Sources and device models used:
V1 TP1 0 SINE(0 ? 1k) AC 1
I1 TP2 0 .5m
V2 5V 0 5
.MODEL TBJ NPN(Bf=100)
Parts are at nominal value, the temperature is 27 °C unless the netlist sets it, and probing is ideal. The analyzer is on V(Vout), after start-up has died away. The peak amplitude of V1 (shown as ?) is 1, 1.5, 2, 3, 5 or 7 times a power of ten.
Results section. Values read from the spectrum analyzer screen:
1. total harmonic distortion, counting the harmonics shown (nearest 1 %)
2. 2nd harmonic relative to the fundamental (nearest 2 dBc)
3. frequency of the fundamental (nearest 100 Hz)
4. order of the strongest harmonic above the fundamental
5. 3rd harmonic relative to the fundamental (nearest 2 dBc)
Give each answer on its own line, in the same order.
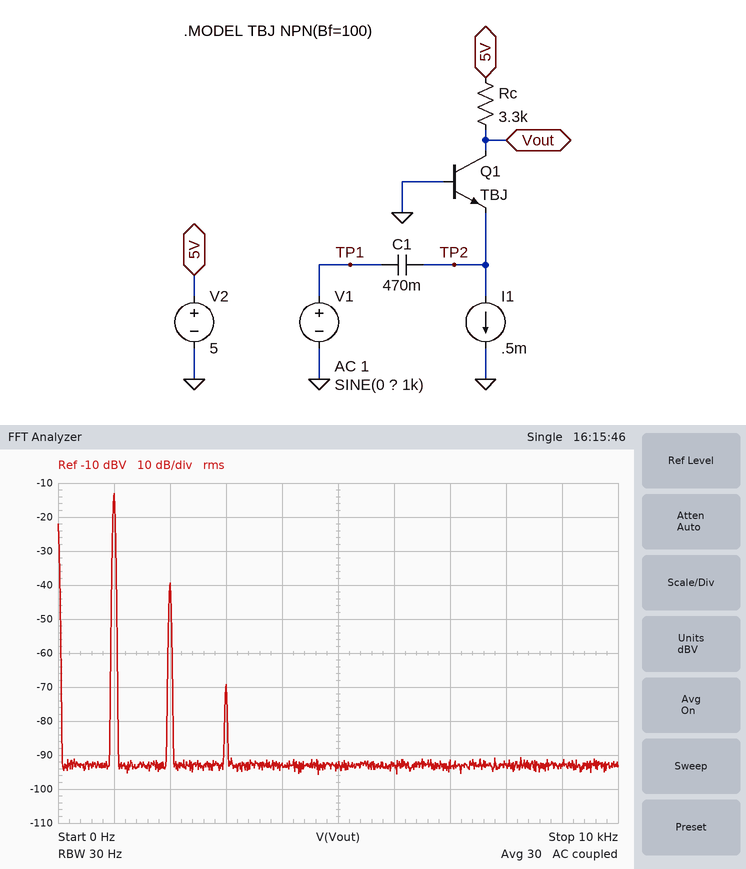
5 %
-26 dBc
1.0 kHz
2
-56 dBc
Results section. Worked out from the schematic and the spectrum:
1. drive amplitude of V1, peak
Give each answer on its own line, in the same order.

5 mV
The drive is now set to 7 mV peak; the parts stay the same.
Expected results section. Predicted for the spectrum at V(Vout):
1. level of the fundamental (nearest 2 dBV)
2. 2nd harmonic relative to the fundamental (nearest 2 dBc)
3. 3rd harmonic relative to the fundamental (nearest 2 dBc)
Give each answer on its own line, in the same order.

-10 dBV
-24 dBc
-50 dBc
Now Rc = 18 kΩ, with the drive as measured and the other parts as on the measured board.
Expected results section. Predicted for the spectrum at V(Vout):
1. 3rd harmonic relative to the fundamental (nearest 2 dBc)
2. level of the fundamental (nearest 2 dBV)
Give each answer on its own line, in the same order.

-48 dBc
-44 dBV
